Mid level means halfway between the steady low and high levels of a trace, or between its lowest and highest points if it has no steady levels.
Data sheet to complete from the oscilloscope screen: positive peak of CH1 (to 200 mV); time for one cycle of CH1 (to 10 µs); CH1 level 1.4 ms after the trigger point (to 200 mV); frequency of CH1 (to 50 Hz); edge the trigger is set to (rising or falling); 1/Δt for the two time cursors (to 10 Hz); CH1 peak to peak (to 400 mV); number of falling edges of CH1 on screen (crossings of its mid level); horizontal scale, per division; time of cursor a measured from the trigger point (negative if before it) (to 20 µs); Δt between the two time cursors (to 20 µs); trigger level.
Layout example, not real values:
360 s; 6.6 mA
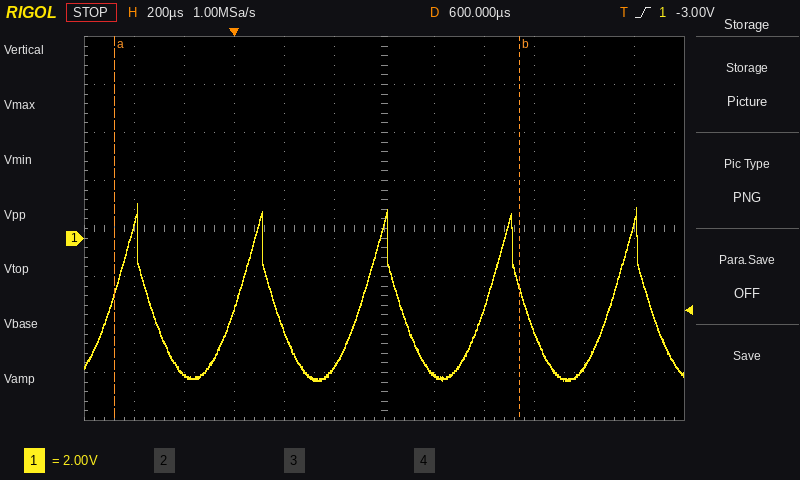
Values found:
1.4 V; 500 µs; -5.4 V; 2.00 kHz; rising; 620 Hz; 7.2 V; 5; 200 µs; -480 µs; 1.62 ms; -3.00 V
